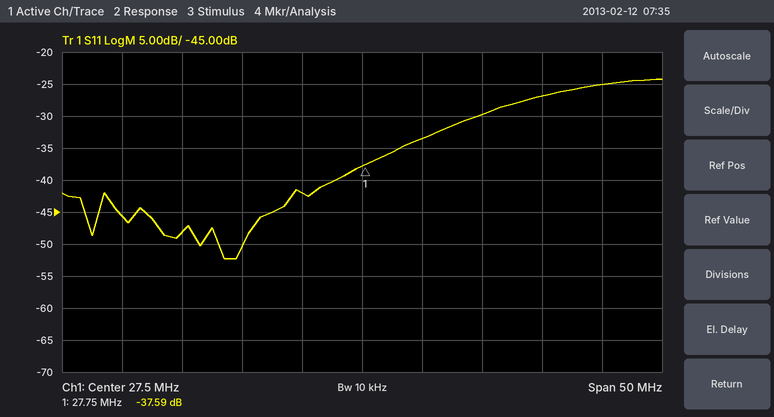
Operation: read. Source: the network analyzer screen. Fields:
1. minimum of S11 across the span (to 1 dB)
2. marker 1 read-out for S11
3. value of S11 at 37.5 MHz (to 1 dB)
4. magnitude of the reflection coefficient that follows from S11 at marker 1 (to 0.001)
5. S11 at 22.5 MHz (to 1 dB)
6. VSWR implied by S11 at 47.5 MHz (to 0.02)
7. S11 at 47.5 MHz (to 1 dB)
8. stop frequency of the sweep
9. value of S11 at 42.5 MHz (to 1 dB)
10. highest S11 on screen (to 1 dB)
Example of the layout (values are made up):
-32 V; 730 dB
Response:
-52 dB; -37.59 dB; -30 dB; 0.013; -42 dB; 1.12; -25 dB; 52.5 MHz; -27 dB; -24 dB
